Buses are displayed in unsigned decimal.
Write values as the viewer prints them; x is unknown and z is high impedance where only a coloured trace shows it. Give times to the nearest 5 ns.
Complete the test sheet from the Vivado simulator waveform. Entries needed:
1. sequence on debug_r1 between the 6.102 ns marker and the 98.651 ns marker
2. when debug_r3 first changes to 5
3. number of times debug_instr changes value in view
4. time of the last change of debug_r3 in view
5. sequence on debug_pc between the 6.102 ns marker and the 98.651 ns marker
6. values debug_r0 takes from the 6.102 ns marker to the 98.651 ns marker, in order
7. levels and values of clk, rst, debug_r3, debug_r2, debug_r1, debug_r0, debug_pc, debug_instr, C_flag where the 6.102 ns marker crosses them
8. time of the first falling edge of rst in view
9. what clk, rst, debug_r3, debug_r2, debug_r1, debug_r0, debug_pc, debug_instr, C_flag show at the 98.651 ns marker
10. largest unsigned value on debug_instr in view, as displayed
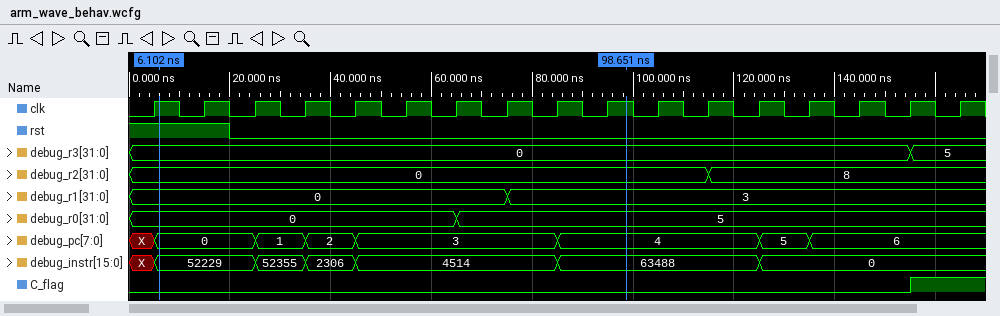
0, 3
155 ns
6
155 ns
0, 1, 2, 3, 4
0, 5
clk=1, rst=1, debug_r3=0, debug_r2=0, debug_r1=0, debug_r0=0, debug_pc=0, debug_instr=52229, C_flag=0
20 ns
clk=1, rst=0, debug_r3=0, debug_r2=0, debug_r1=3, debug_r0=5, debug_pc=4, debug_instr=63488, C_flag=0
63488
